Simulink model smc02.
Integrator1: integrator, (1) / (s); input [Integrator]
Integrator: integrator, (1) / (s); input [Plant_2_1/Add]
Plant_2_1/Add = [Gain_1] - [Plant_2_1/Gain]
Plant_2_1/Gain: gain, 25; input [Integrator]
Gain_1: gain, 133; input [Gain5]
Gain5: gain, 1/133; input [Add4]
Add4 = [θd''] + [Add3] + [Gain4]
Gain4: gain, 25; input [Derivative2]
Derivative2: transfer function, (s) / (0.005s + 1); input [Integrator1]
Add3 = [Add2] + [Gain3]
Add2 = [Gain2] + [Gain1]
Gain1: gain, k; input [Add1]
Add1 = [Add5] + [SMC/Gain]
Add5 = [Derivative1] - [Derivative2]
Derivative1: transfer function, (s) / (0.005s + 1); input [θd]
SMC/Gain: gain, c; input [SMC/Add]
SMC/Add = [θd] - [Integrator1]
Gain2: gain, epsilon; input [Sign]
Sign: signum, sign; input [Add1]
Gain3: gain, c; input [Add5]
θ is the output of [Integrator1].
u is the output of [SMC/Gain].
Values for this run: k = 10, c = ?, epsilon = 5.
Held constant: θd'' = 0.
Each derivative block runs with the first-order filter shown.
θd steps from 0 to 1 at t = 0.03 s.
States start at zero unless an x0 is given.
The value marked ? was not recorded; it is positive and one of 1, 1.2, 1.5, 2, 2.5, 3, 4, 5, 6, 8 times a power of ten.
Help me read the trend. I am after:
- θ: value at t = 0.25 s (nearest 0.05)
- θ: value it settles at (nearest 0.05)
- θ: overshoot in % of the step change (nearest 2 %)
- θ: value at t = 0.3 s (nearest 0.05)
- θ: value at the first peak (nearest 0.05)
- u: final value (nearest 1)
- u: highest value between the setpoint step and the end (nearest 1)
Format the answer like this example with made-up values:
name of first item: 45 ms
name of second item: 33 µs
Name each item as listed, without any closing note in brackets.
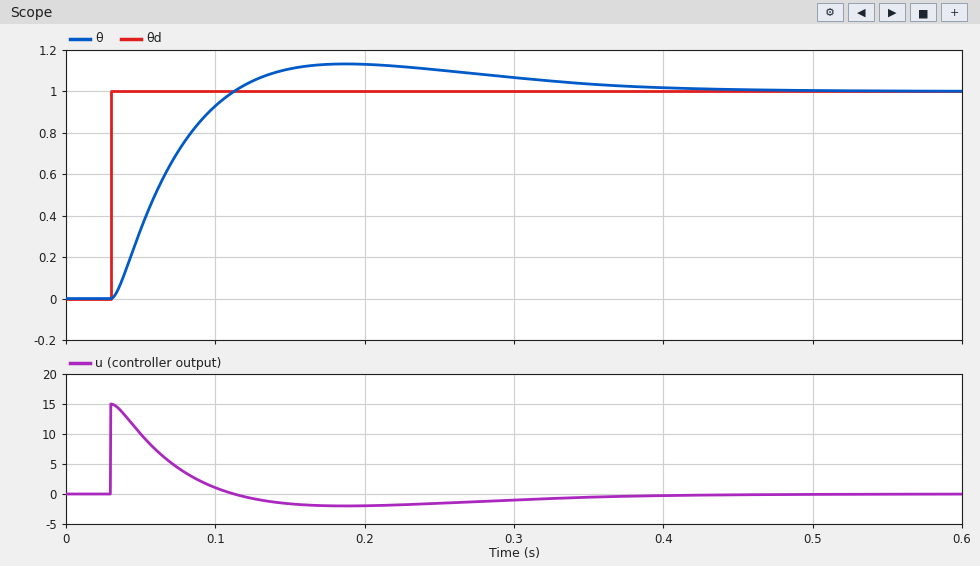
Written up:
θ: value at t = 0.25 s: 1.10
θ: value it settles at: 1.00
θ: overshoot in % of the step change: 14 %
θ: value at t = 0.3 s: 1.05
θ: value at the first peak: 1.15
u: final value: 0
u: highest value between the setpoint step and the end: 15
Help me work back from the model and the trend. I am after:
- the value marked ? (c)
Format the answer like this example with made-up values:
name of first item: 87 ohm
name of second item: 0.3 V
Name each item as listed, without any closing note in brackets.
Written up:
the value marked ?: 15
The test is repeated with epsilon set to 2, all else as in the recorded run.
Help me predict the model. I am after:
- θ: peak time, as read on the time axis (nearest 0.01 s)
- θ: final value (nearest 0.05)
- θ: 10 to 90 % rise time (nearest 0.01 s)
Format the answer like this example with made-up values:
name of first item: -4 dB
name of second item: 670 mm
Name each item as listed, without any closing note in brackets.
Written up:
θ: peak time, as read on the time axis: 0.19 s
θ: final value: 1.00
θ: 10 to 90 % rise time: 0.06 s
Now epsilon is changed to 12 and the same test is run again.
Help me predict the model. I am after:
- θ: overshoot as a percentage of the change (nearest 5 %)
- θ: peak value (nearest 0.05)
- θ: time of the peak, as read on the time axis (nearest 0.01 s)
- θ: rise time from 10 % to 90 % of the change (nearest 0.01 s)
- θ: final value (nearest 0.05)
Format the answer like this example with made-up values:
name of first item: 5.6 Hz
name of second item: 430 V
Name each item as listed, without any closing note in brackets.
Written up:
θ: overshoot as a percentage of the change: 10 %
θ: peak value: 1.10
θ: time of the peak, as read on the time axis: 0.18 s
θ: rise time from 10 % to 90 % of the change: 0.06 s
θ: final value: 1.00
